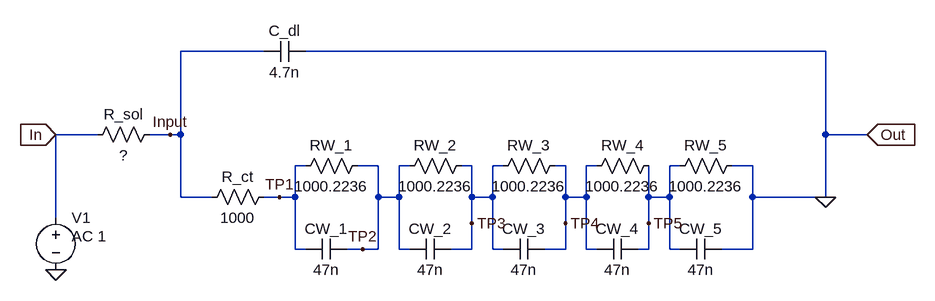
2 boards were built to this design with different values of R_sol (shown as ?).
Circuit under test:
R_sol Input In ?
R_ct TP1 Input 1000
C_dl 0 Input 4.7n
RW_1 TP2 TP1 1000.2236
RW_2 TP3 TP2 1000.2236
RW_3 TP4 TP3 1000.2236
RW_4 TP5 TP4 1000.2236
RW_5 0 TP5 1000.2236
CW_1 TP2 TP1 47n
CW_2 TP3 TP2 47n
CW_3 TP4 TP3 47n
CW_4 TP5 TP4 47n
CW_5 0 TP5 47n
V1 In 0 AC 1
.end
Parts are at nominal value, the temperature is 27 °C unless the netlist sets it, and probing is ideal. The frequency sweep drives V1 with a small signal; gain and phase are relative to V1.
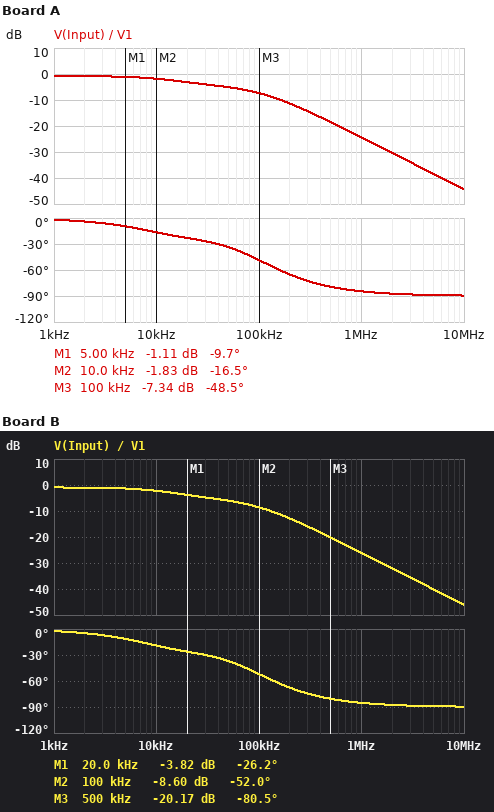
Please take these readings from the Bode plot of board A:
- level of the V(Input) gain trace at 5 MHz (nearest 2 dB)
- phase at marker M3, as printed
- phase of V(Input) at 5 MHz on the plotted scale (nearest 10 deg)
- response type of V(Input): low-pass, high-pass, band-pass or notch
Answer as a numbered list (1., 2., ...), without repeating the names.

1. -38 dB
2. -48.5 deg
3. -90 deg
4. low-pass
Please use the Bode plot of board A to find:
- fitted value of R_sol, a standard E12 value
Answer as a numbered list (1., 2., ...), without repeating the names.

1. 560 Ω
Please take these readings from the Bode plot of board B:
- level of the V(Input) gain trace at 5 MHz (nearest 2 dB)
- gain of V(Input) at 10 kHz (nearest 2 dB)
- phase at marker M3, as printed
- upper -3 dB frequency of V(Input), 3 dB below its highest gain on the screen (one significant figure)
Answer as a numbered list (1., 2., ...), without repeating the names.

1. -40 dB
2. -2 dB
3. -80.5 deg
4. 20 kHz
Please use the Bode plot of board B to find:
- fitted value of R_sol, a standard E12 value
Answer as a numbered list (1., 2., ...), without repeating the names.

1. 680 Ω
